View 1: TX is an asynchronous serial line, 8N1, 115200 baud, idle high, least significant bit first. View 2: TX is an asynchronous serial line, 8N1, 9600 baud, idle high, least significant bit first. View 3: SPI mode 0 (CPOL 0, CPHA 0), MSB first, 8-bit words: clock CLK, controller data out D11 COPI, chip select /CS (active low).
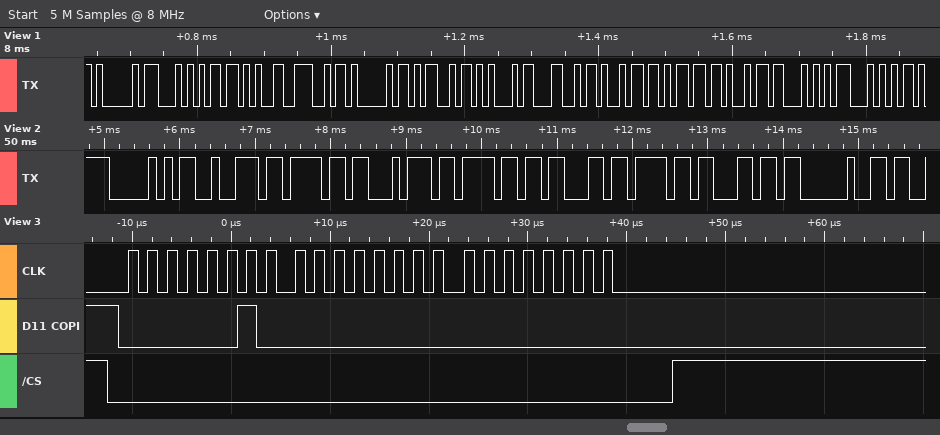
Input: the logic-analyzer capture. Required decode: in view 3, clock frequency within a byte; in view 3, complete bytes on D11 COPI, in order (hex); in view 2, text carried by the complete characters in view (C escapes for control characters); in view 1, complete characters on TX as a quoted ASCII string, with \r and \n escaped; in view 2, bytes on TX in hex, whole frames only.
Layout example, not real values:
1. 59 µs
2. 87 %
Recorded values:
1. 500 kHz
2. 02 00 00
3. "Protocol "
4. "AT+NAMELimiTT"
5. 0x50 0x72 0x6F 0x74 0x6F 0x63 0x6F 0x6C 0x20
